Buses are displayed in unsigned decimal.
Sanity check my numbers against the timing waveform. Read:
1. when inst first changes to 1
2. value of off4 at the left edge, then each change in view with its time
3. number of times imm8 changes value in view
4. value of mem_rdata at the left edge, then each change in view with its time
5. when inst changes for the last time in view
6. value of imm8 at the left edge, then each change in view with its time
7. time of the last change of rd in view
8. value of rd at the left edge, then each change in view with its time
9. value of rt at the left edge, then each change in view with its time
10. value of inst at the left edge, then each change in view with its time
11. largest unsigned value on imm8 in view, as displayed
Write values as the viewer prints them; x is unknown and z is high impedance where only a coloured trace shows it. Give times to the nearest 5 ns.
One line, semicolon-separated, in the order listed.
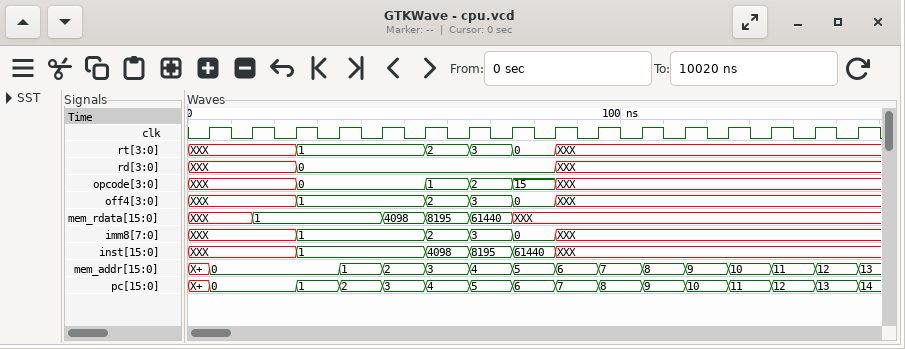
25 ns; XXX, 1 at 25 ns, 2 at 55 ns, 3 at 65 ns, 0 at 75 ns, XXX at 85 ns; 5; XXX, 1 at 15 ns, 4098 at 45 ns, 8195 at 55 ns, 61440 at 65 ns, XXX at 75 ns; 85 ns; XXX, 1 at 25 ns, 2 at 55 ns, 3 at 65 ns, 0 at 75 ns, XXX at 85 ns; 85 ns; XXX, 0 at 25 ns, XXX at 85 ns; XXX, 1 at 25 ns, 2 at 55 ns, 3 at 65 ns, 0 at 75 ns, XXX at 85 ns; XXX, 1 at 25 ns, 4098 at 55 ns, 8195 at 65 ns, 61440 at 75 ns, XXX at 85 ns; 3
